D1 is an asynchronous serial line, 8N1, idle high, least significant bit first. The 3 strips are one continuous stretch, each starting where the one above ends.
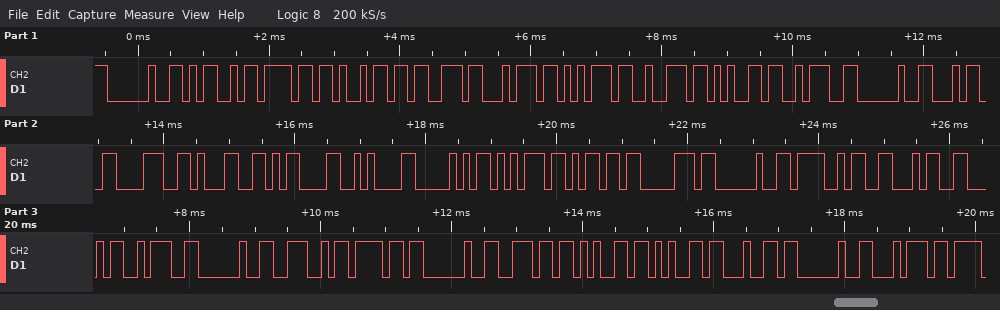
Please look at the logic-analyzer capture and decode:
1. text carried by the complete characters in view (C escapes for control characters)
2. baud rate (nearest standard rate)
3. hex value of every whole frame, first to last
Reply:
" Moisture: 481\r\nPump OFF: No need t"
9600 baud
20 4D 6F 69 73 74 75 72 65 3A 20 34 38 31 0D 0A 50 75 6D 70 20 4F 46 46 3A 20 4E 6F 20 6E 65 65 64 20 74
